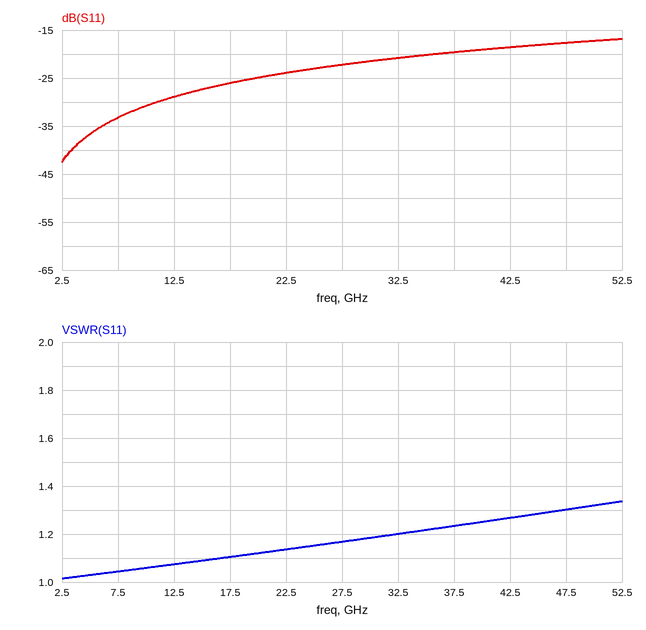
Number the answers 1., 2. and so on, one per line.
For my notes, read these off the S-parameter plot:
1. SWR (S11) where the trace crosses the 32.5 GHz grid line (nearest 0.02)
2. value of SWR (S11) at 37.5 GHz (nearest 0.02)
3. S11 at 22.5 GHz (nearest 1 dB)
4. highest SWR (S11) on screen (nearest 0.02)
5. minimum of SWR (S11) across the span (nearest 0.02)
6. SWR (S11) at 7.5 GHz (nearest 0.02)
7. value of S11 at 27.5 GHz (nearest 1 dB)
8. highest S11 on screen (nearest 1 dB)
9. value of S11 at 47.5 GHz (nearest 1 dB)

1. 1.20
2. 1.24
3. -24 dB
4. 1.34
5. 1.02
6. 1.04
7. -22 dB
8. -17 dB
9. -18 dB
